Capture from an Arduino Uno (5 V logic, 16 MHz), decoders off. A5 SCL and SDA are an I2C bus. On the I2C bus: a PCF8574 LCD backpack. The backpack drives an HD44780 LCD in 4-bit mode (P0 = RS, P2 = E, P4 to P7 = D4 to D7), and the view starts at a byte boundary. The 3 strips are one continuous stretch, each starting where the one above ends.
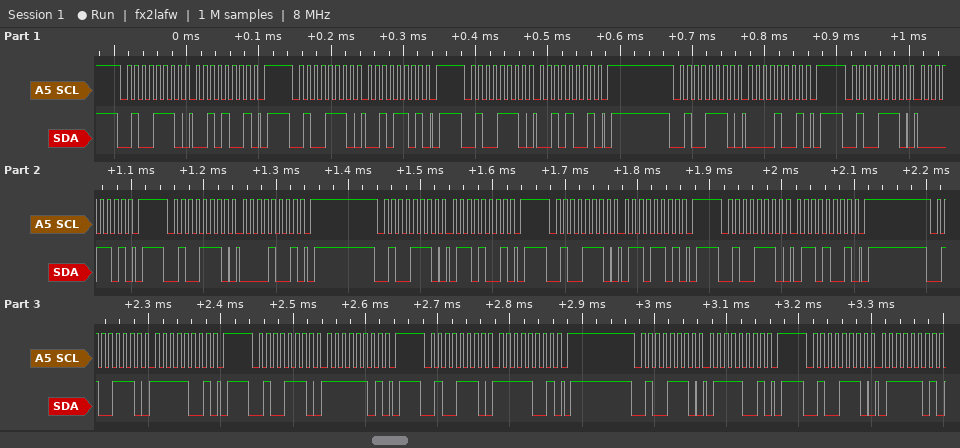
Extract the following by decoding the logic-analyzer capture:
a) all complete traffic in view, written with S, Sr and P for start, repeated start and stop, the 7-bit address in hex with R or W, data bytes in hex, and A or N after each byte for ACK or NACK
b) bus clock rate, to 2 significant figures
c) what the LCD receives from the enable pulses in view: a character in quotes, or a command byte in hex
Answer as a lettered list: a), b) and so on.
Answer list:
a) S 27W A 29 A P S 27W A 2D A P S 27W A 29 A P S 27W A 09 A P S 27W A 0D A P S 27W A 09 A P S 27W A 69 A P S 27W A 6D A P S 27W A 69 A P S 27W A F9 A P S 27W A FD A P S 27W A F9 A P S 27W A 79 A P S 27W A 7D A
b) 100 kHz
c) ' ' 'o'
